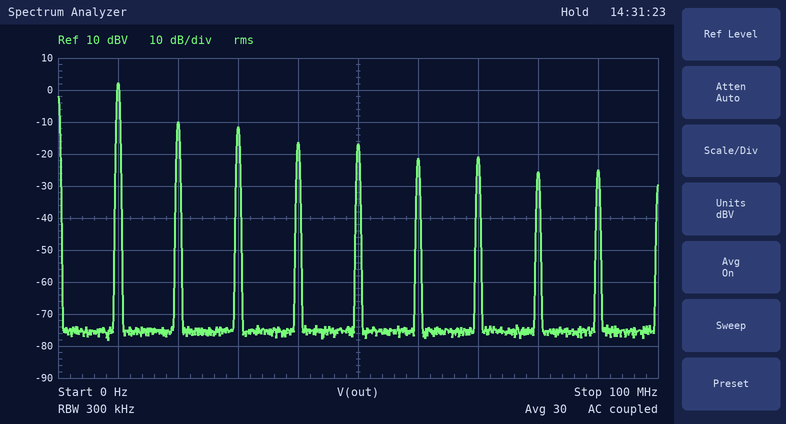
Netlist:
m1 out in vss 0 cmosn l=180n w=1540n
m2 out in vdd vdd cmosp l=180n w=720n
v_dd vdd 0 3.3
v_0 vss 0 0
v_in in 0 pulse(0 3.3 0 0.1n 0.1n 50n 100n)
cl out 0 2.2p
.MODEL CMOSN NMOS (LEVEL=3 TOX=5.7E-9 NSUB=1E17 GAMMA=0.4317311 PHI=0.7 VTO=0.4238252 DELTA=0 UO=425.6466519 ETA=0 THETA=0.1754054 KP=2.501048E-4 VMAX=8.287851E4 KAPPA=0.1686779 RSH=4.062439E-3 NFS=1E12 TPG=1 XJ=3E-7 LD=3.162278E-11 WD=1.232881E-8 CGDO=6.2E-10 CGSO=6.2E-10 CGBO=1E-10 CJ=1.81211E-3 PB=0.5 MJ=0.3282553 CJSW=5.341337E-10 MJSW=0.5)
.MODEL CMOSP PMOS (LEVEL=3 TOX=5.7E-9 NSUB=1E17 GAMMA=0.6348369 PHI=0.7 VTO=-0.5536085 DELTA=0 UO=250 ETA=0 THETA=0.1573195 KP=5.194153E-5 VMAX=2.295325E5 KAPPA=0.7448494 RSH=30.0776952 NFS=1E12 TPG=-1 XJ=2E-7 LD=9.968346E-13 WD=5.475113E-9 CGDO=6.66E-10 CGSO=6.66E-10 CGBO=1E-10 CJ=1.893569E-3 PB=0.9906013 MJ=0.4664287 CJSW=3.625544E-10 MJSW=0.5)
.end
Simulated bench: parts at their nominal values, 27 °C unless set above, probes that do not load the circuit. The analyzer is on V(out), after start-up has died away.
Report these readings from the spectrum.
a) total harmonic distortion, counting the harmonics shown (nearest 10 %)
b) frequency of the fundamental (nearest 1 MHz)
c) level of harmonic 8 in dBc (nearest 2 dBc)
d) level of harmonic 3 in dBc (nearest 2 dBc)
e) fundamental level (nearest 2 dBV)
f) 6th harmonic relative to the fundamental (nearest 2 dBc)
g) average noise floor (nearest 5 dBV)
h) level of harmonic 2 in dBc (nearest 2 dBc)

40 %
10 MHz
-28 dBc
-14 dBc
2 dBV
-24 dBc
-75 dBV
-12 dBc
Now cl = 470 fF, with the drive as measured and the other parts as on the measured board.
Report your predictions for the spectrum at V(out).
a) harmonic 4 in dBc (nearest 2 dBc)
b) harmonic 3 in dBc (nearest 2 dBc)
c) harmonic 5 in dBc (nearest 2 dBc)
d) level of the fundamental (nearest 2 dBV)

-24 dBc
-10 dBc
-16 dBc
4 dBV
